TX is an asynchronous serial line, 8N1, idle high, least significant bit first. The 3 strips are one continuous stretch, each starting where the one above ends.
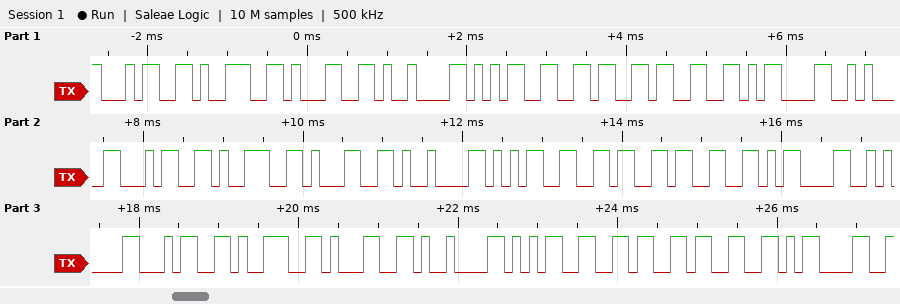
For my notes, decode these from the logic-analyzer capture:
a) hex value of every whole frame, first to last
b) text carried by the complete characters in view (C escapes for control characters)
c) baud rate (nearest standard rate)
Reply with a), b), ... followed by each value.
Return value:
a) 34 39 31 09 35 36 33 0D 0A 34 39 31 09 35 36 33 0D 0A 34 39 31 09 35 36 33 0D
b) "491\t563\r\n491\t563\r\n491\t563\r"
c) 9600 baud
